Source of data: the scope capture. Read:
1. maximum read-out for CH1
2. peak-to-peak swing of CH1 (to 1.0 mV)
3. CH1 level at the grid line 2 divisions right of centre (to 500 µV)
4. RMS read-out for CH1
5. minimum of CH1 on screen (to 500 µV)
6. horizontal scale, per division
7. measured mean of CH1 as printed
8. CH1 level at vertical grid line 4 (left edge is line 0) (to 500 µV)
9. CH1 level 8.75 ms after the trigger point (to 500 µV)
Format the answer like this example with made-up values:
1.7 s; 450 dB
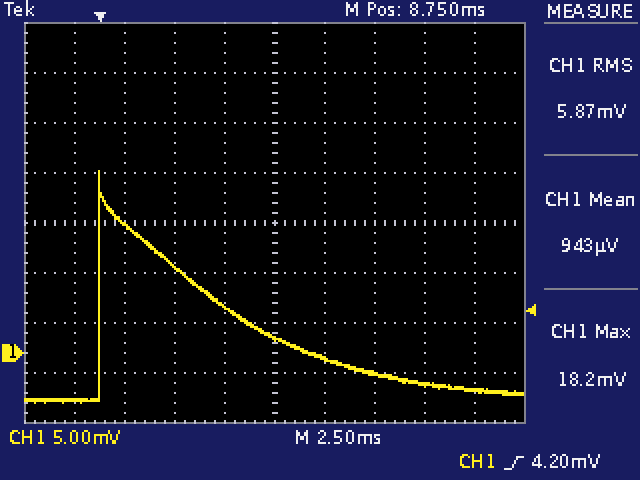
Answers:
18.2 mV; 23.0 mV; -2.0 mV; 5.87 mV; -5.0 mV; 2.5 ms; 943 µV; 4.5 mV; 1.5 mV
